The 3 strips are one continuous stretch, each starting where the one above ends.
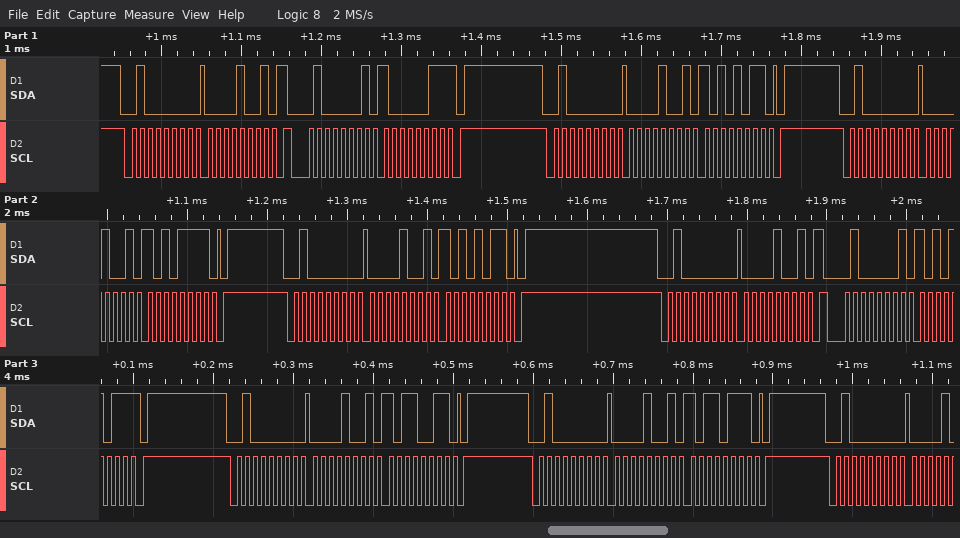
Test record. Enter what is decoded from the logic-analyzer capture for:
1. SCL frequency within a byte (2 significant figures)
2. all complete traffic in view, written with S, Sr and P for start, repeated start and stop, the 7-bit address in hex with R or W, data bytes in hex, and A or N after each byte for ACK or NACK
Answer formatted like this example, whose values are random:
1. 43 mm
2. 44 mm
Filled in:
1. 100 kHz
2. S 20W A 09 A Sr 20R A 83 N P S 20W A 09 A AB A P S 20W A 09 A AF A P S 20W A 09 A AB A P S 20W A 09 A Sr 20R A AB N P S 20W A 09 A B3 A P S 20W A 09 A B7 A P S 20W A
